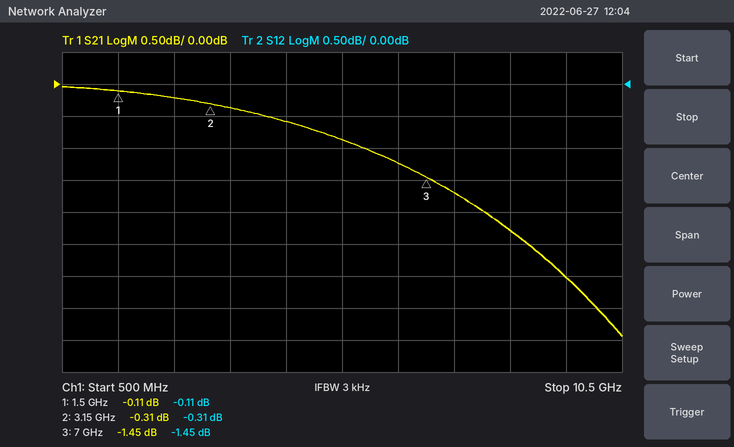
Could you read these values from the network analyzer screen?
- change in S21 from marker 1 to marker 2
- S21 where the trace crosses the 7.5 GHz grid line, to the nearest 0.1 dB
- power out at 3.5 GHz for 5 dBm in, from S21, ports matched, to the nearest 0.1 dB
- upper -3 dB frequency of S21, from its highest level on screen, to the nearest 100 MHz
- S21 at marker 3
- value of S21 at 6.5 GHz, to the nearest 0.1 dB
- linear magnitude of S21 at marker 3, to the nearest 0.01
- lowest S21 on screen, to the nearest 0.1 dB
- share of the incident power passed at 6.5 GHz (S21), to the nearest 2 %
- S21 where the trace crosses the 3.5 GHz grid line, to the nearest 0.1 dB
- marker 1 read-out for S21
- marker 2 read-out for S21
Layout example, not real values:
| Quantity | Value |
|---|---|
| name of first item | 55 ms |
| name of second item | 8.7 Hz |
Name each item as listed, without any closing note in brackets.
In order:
| Quantity | Value |
|---|---|
| change in S21 from marker 1 to marker 2 | -0.20 dB |
| S21 where the trace crosses the 7.5 GHz grid line, to the nearest 0.1 dB | -1.7 dB |
| power out at 3.5 GHz for 5 dBm in, from S21, ports matched, to the nearest 0.1 dB | 4.6 dBm |
| upper -3 dB frequency of S21, from its highest level on screen, to the nearest 100 MHz | 9.5 GHz |
| S21 at marker 3 | -1.45 dB |
| value of S21 at 6.5 GHz, to the nearest 0.1 dB | -1.2 dB |
| linear magnitude of S21 at marker 3, to the nearest 0.01 | 0.85 |
| lowest S21 on screen, to the nearest 0.1 dB | -3.9 dB |
| share of the incident power passed at 6.5 GHz (S21), to the nearest 2 % | 76 % |
| S21 where the trace crosses the 3.5 GHz grid line, to the nearest 0.1 dB | -0.4 dB |
| marker 1 read-out for S21 | -0.11 dB |
| marker 2 read-out for S21 | -0.31 dB |
